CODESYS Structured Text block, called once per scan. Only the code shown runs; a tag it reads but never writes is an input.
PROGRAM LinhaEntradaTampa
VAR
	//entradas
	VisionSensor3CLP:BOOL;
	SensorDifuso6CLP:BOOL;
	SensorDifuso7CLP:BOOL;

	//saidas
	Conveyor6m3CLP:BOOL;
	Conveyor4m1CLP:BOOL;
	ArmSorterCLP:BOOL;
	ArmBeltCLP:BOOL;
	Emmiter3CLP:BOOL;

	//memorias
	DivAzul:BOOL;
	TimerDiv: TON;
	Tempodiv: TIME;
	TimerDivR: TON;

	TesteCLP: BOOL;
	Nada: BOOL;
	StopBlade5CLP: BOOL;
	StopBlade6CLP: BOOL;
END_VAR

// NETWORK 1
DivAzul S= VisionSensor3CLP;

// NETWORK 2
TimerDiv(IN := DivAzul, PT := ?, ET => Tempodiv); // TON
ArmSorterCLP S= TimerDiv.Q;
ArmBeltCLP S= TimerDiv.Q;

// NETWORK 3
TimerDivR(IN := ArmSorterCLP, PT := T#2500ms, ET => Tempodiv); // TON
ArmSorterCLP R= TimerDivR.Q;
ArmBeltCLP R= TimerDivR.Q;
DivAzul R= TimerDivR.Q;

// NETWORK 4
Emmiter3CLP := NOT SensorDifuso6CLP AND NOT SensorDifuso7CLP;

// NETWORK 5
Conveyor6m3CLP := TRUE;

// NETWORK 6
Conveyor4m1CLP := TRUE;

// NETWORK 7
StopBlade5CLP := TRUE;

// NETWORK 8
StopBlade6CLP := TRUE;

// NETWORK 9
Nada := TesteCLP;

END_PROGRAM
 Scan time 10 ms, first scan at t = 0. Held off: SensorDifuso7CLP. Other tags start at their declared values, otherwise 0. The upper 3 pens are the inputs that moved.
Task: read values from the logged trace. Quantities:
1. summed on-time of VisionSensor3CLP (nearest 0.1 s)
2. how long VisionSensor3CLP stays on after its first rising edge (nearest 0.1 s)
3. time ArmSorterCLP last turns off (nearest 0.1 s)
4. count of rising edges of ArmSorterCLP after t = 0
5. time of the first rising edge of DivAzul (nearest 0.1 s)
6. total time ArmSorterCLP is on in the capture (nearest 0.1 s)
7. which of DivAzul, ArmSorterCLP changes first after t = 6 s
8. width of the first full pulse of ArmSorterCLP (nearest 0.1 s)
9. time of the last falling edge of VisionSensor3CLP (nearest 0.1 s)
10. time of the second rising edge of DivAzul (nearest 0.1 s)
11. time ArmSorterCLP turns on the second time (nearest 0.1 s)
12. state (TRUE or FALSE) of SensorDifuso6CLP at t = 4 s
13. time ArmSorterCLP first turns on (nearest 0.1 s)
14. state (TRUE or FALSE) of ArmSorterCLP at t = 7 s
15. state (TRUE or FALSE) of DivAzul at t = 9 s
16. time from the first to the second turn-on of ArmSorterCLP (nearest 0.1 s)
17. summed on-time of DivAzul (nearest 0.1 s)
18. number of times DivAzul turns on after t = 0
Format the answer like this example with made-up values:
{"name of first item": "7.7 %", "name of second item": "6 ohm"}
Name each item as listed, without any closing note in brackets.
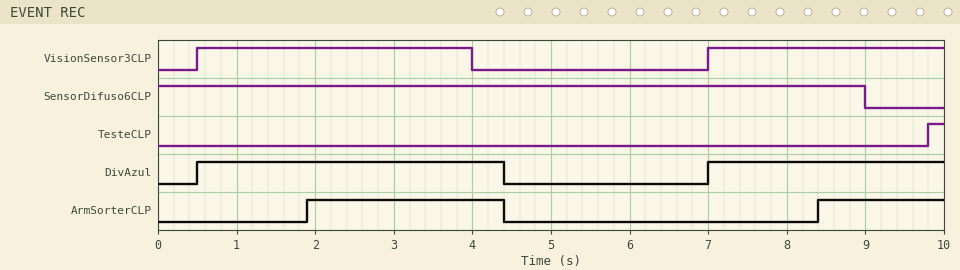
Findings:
{"summed on-time of VisionSensor3CLP": "6.5 s", "how long VisionSensor3CLP stays on after its first rising edge": "3.5 s", "time ArmSorterCLP last turns off": "4.4 s", "count of rising edges of ArmSorterCLP after t = 0": "2", "time of the first rising edge of DivAzul": "0.5 s", "total time ArmSorterCLP is on in the capture": "4.1 s", "which of DivAzul, ArmSorterCLP changes first after t = 6 s": "DivAzul", "width of the first full pulse of ArmSorterCLP": "2.5 s", "time of the last falling edge of VisionSensor3CLP": "4.0 s", "time of the second rising edge of DivAzul": "7.0 s", "time ArmSorterCLP turns on the second time": "8.4 s", "state (TRUE or FALSE) of SensorDifuso6CLP at t = 4 s": "TRUE", "time ArmSorterCLP first turns on": "1.9 s", "state (TRUE or FALSE) of ArmSorterCLP at t = 7 s": "FALSE", "state (TRUE or FALSE) of DivAzul at t = 9 s": "TRUE", "time from the first to the second turn-on of ArmSorterCLP": "6.5 s", "summed on-time of DivAzul": "6.9 s", "number of times DivAzul turns on after t = 0": "2"}
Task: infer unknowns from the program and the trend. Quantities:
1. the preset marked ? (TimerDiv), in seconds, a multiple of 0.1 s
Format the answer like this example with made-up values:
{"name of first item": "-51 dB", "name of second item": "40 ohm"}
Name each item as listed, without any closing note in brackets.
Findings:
{"the preset marked ? (TimerDiv), in seconds, a multiple of 0.1 s": "1.4 s"}
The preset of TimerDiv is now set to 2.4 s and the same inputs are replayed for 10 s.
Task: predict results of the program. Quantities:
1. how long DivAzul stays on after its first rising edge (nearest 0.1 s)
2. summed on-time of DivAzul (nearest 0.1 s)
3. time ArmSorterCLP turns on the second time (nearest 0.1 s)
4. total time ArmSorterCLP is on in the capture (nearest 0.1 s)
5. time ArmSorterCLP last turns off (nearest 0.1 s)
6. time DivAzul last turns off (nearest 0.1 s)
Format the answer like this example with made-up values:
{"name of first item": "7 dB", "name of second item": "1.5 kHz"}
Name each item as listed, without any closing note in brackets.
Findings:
{"how long DivAzul stays on after its first rising edge": "4.9 s", "summed on-time of DivAzul": "7.9 s", "time ArmSorterCLP turns on the second time": "9.4 s", "total time ArmSorterCLP is on in the capture": "3.1 s", "time ArmSorterCLP last turns off": "5.4 s", "time DivAzul last turns off": "5.4 s"}
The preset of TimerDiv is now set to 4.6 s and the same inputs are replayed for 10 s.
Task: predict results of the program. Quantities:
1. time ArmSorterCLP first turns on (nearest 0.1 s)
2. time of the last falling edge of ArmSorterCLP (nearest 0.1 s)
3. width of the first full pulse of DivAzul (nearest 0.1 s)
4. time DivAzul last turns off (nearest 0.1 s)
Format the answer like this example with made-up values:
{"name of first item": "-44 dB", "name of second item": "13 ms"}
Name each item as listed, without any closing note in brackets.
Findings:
{"time ArmSorterCLP first turns on": "5.1 s", "time of the last falling edge of ArmSorterCLP": "7.6 s", "width of the first full pulse of DivAzul": "7.1 s", "time DivAzul last turns off": "7.6 s"}
